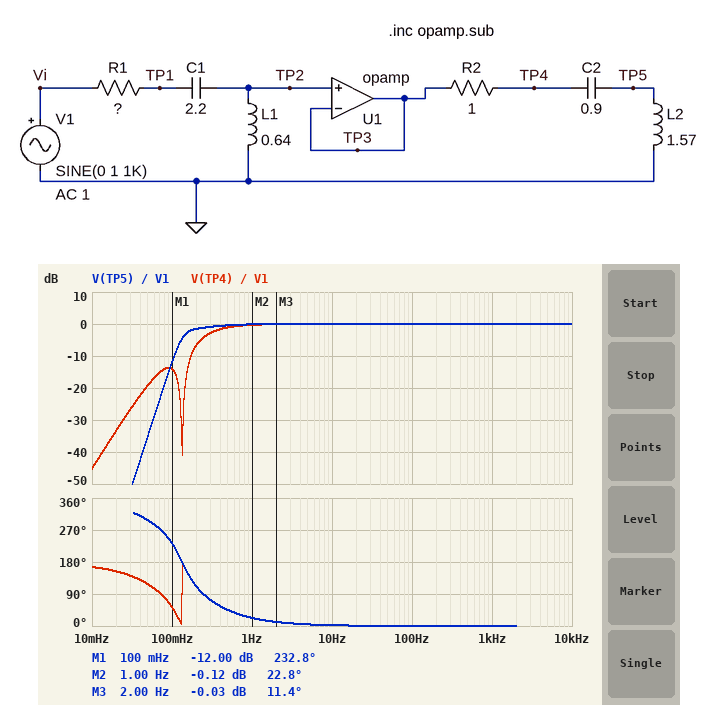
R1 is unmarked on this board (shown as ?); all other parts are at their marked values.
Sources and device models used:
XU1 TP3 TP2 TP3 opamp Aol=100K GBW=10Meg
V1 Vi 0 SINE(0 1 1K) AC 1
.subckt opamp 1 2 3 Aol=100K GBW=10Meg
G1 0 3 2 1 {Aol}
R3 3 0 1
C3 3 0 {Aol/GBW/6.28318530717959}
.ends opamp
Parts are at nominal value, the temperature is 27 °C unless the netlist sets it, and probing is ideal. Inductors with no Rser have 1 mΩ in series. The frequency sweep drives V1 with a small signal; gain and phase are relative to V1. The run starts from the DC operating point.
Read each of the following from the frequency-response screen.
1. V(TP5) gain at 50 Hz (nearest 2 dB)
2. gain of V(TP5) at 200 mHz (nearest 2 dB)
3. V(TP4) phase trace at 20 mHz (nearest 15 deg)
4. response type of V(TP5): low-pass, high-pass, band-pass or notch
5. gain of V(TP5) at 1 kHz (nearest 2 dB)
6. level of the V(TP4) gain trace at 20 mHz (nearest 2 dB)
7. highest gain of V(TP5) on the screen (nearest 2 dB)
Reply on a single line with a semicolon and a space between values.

0 dB; -2 dB; 150 deg; high-pass; 0 dB; -34 dB; 0 dB
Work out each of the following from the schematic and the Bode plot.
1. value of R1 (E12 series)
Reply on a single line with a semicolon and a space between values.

1.2 Ω
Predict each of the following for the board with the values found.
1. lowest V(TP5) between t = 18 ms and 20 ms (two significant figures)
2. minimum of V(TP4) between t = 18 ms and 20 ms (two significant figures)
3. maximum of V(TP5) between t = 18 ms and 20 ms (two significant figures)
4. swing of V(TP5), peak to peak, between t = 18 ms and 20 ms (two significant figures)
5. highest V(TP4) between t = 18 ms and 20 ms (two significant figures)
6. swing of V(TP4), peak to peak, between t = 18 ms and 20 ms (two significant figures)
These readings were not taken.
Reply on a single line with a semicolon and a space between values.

-1.0 V; -1.0 V; 1.0 V; 2.0 V; 1.0 V; 2.0 V
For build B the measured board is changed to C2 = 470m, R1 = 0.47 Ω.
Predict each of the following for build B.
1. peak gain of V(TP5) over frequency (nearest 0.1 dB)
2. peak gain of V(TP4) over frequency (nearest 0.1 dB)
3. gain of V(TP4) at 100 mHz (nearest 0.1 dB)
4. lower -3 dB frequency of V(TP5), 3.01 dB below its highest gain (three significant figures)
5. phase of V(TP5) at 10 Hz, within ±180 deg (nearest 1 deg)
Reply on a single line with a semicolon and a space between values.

7.5 dB; 0.2 dB; -3.7 dB; 157 mHz; 1 deg
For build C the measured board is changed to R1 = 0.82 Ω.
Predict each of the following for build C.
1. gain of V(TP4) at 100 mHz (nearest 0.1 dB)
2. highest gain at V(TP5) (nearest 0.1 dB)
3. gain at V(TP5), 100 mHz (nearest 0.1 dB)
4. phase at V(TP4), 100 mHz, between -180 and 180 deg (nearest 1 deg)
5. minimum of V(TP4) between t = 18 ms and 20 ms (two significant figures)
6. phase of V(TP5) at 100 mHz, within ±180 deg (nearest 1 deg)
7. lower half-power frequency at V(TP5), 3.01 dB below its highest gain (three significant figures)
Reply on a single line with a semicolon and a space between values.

-11.0 dB; 1.2 dB; -9.0 dB; 59 deg; -1.0 V; -121 deg; 130 mHz
